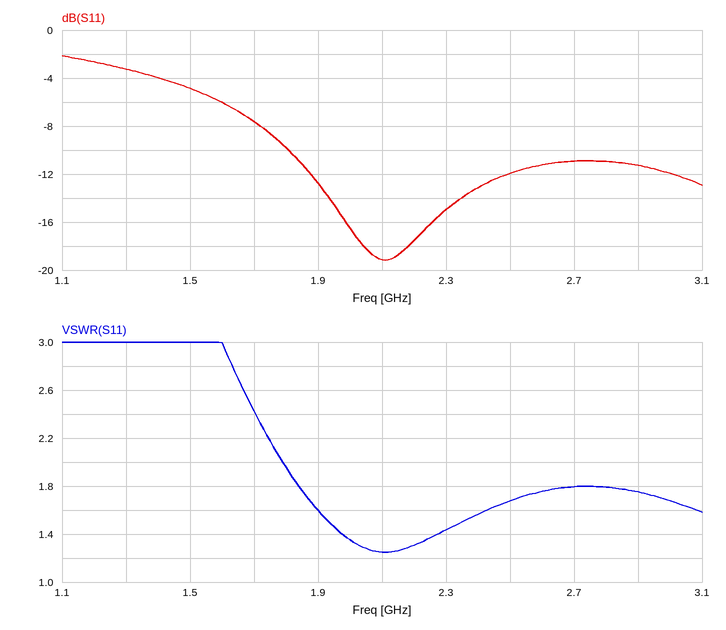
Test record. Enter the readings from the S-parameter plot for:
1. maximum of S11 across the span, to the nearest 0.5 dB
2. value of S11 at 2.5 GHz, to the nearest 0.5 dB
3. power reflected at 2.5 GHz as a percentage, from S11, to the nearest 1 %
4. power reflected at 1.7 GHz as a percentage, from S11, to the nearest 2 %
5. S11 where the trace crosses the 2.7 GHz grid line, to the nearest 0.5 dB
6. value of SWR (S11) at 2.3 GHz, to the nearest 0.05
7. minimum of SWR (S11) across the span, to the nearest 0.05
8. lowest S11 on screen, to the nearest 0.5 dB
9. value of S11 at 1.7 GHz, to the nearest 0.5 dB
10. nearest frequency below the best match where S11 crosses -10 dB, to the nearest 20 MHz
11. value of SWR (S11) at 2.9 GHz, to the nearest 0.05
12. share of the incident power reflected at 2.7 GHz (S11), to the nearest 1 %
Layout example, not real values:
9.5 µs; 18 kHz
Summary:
-2.0 dB; -12.0 dB; 6 %; 18 %; -11.0 dB; 1.45; 1.25; -19.0 dB; -7.5 dB; 1.80 GHz; 1.75; 8 %
